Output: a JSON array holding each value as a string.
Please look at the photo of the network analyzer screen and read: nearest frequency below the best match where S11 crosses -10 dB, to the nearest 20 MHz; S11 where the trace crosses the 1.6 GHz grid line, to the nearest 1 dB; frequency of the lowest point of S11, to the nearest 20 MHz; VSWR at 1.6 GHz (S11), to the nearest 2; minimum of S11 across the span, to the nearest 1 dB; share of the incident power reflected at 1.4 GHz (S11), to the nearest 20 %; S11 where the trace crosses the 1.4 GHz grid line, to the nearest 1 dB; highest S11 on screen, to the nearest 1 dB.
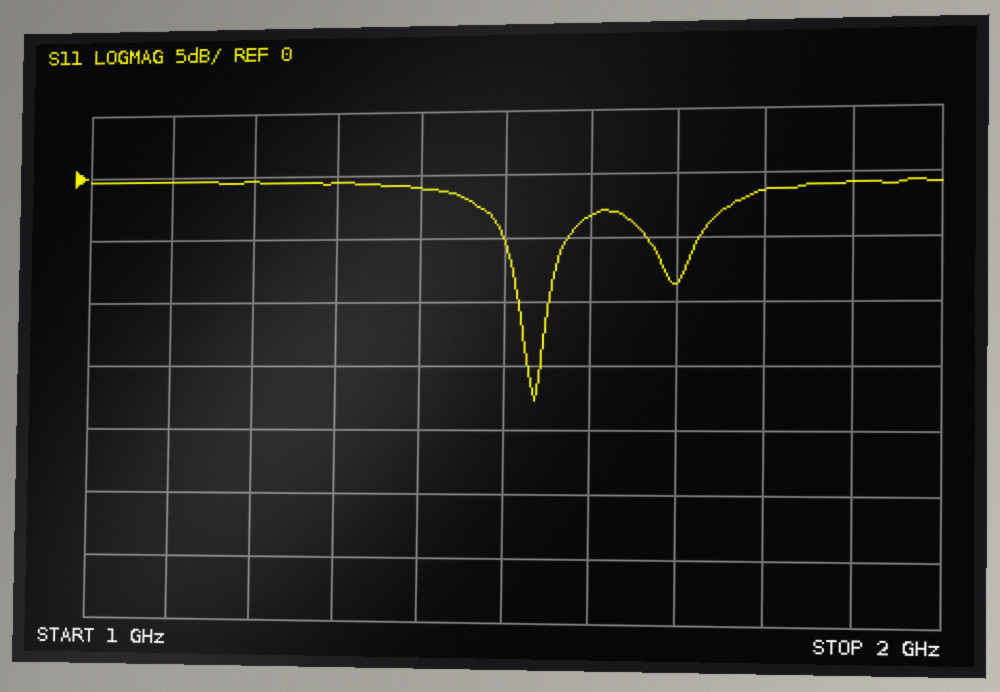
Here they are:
["1.52 GHz", "-3 dB", "1.54 GHz", "6", "-18 dB", "80 %", "-1 dB", "0 dB"]
